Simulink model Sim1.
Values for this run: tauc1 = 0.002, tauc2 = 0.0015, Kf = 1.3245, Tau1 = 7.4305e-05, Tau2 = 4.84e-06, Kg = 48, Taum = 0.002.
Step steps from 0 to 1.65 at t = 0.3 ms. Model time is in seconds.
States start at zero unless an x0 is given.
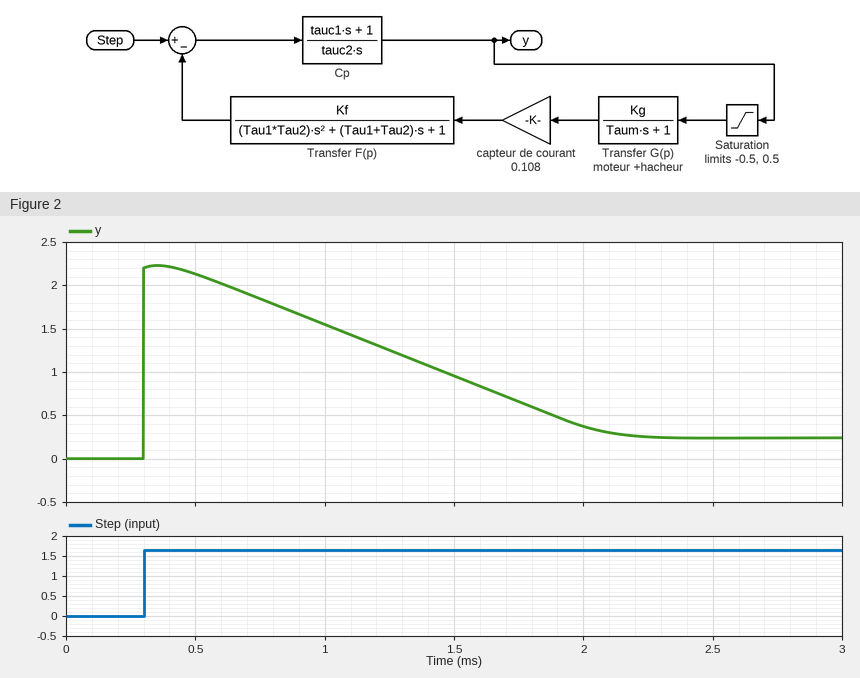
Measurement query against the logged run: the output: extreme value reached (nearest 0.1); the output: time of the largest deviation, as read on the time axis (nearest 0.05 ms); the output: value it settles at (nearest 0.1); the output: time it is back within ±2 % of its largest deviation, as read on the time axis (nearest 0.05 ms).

2.2
0.35 ms
0.2
2.15 ms
